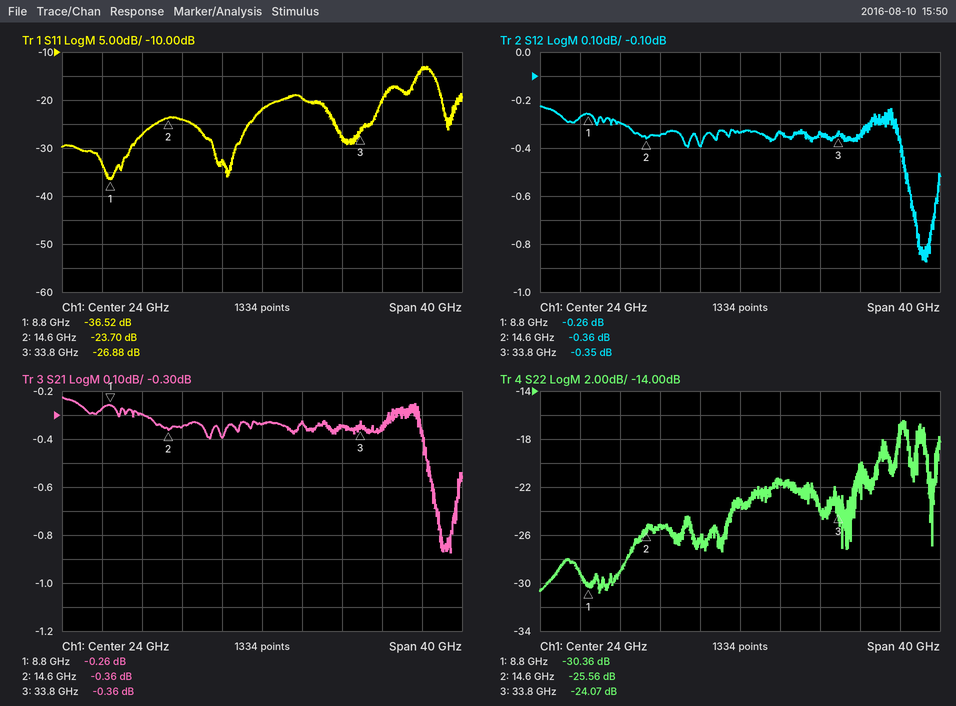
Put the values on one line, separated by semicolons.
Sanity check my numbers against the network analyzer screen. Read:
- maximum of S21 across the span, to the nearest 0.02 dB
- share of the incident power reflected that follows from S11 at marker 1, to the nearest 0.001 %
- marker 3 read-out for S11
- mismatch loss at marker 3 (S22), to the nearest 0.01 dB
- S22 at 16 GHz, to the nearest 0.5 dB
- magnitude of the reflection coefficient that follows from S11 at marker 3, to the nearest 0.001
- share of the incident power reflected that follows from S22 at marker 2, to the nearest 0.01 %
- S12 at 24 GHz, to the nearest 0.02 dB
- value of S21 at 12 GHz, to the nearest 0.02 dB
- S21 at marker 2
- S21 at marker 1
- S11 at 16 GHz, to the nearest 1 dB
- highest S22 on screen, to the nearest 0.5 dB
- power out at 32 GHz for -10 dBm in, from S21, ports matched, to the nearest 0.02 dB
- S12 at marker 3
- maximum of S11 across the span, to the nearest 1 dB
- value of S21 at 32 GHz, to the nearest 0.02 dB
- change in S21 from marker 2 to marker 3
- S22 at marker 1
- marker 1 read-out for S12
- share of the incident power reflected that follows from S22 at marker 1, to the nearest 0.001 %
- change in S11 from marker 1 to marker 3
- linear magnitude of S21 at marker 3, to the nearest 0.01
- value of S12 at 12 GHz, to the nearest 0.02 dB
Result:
-0.22 dB; 0.022 %; -26.88 dB; 0.02 dB; -25.0 dB; 0.045; 0.28 %; -0.34 dB; -0.30 dB; -0.36 dB; -0.26 dB; -24 dB; -16.5 dB; -10.34 dBm; -0.35 dB; -13 dB; -0.34 dB; 0.00 dB; -30.36 dB; -0.26 dB; 0.092 %; 9.64 dB; 0.96; -0.30 dB
